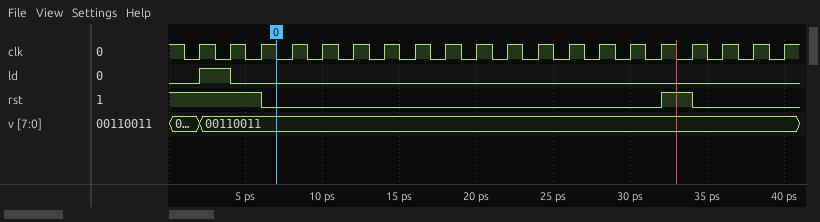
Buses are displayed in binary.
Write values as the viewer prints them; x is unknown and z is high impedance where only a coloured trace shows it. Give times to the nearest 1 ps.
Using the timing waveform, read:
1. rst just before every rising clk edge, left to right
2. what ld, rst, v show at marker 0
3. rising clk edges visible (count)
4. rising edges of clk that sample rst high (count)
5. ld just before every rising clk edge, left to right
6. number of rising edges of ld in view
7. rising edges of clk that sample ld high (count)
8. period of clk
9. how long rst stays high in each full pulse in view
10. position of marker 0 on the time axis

1 1 1 0 0 0 0 0 0 0 0 0 0 0 0 0 1 0 0 0
ld=0, rst=0, v=00110011
20
4
0 1 0 0 0 0 0 0 0 0 0 0 0 0 0 0 0 0 0 0
1
1
2 ps
2 ps
7 ps
